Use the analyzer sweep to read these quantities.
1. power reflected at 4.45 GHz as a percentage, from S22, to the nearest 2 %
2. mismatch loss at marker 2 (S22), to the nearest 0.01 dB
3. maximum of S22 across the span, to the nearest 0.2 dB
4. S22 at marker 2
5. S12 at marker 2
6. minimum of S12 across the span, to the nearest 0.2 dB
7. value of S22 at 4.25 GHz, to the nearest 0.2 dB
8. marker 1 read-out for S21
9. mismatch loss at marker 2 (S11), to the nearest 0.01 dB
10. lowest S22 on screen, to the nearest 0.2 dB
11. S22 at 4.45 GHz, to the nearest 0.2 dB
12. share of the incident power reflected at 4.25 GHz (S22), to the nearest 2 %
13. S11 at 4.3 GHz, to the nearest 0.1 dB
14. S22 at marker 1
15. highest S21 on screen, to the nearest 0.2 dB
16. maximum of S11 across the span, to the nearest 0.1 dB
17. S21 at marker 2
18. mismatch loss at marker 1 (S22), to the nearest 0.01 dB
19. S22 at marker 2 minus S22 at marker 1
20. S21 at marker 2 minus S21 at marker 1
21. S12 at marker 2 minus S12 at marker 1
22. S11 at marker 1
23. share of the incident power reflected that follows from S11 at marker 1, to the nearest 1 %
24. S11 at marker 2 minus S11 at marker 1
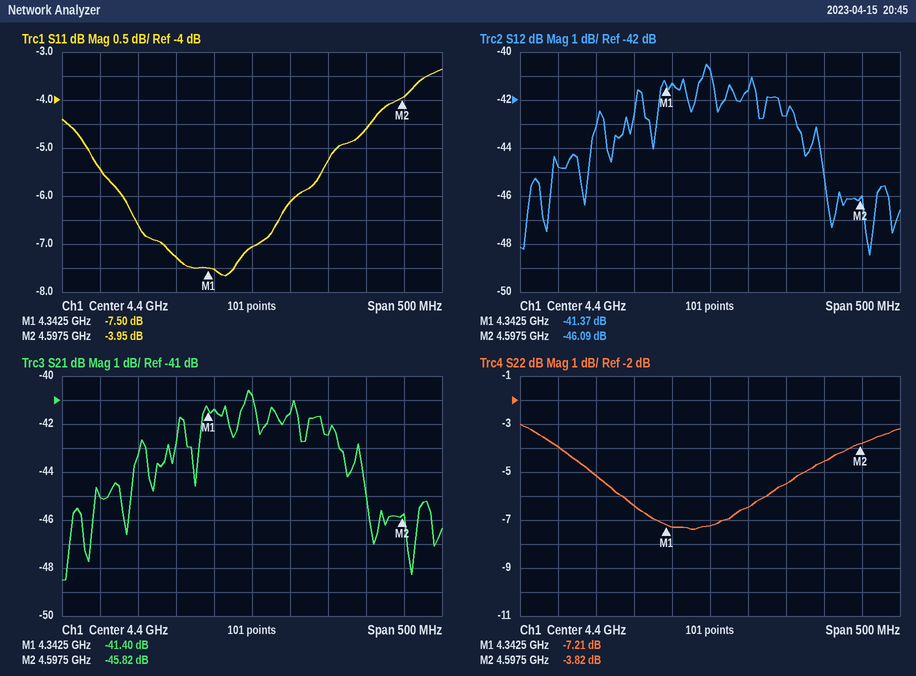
22 %
2.33 dB
-3.0 dB
-3.82 dB
-46.09 dB
-48.4 dB
-5.2 dB
-41.40 dB
2.24 dB
-7.4 dB
-6.4 dB
30 %
-7.3 dB
-7.21 dB
-40.6 dB
-3.4 dB
-45.82 dB
0.92 dB
3.39 dB
-4.42 dB
-4.72 dB
-7.50 dB
18 %
3.55 dB
